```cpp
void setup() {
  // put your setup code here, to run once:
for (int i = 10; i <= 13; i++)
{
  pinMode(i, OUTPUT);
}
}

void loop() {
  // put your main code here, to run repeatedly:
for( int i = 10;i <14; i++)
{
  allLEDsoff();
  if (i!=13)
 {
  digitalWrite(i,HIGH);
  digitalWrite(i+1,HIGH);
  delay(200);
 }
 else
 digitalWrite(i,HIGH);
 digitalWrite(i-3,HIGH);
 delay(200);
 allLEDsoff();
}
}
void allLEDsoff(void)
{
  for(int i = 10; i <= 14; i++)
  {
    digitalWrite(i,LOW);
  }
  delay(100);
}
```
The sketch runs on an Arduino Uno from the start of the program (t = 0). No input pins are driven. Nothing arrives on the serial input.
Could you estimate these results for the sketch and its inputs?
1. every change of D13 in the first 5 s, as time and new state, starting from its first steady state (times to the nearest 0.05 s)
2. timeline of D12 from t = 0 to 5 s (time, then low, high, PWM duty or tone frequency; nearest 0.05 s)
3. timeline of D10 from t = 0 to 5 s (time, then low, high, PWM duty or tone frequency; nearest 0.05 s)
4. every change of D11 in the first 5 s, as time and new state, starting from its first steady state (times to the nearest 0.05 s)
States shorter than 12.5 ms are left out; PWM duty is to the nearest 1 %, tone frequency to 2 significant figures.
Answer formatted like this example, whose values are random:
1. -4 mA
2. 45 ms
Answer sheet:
1. 0 s low; 1.3 s high; 1.7 s low; 1.9 s high; 2.1 s low; 3.5 s high; 3.9 s low; 4.1 s high; 4.3 s low
2. 0 s low; 0.7 s high; 1.1 s low; 1.3 s high; 1.7 s low; 2.9 s high; 3.3 s low; 3.5 s high; 3.9 s low
3. 0 s low; 0.1 s high; 0.5 s low; 1.9 s high; 2.1 s low; 2.3 s high; 2.7 s low; 4.1 s high; 4.3 s low; 4.5 s high; 4.9 s low
4. 0 s low; 0.1 s high; 0.5 s low; 0.7 s high; 1.1 s low; 2.3 s high; 2.7 s low; 2.9 s high; 3.3 s low; 4.5 s high; 4.9 s low
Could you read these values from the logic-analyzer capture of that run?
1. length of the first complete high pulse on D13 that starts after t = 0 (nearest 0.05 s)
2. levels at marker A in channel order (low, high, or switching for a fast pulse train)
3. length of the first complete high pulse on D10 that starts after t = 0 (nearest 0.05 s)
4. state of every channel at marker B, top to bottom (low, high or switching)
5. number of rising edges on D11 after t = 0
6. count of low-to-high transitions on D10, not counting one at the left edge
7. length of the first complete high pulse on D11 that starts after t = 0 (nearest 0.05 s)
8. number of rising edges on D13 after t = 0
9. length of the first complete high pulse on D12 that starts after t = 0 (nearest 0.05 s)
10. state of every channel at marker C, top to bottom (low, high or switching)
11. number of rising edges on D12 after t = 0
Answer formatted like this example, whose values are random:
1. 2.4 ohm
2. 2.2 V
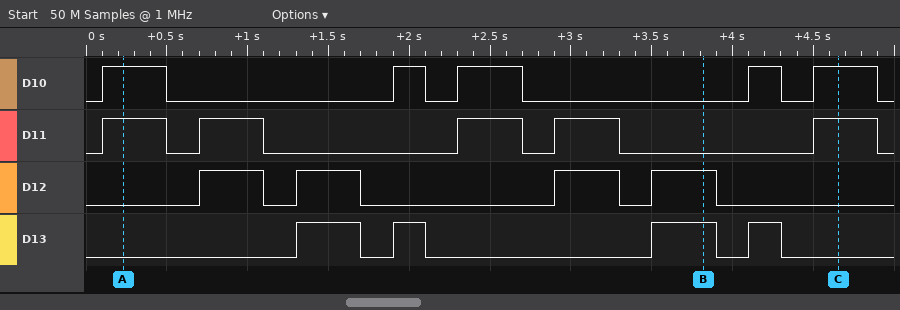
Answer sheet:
1. 0.40 s
2. D10 high, D11 high, D12 low, D13 low
3. 0.40 s
4. D10 low, D11 low, D12 high, D13 high
5. 5
6. 5
7. 0.40 s
8. 4
9. 0.40 s
10. D10 high, D11 high, D12 low, D13 low
11. 4
